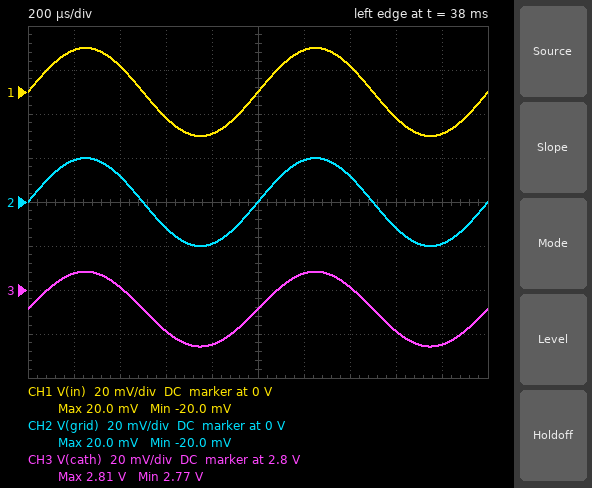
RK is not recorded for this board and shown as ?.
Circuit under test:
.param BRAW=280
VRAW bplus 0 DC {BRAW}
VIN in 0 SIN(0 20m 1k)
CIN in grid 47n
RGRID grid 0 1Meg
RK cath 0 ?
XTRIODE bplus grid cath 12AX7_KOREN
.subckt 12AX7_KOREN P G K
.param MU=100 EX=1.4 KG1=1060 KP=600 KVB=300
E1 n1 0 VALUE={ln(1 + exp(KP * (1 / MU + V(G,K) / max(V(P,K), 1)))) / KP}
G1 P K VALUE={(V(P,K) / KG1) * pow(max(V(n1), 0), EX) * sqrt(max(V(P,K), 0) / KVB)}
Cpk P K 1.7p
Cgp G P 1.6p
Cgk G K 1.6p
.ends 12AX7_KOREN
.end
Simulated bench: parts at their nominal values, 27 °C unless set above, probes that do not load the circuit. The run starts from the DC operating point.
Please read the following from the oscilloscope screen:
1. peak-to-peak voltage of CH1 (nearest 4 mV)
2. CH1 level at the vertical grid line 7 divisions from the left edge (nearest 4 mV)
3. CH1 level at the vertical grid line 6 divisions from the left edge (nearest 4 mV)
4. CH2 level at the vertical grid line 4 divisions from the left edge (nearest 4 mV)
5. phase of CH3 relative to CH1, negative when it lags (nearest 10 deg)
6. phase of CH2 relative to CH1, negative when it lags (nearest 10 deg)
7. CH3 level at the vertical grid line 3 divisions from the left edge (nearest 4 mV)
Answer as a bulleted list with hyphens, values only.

- 40 mV
- 12 mV
- 20 mV
- -20 mV
- 0 deg
- 0 deg
- 2.780 V
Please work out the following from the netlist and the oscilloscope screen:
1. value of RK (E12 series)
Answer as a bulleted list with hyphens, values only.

- 150 kΩ
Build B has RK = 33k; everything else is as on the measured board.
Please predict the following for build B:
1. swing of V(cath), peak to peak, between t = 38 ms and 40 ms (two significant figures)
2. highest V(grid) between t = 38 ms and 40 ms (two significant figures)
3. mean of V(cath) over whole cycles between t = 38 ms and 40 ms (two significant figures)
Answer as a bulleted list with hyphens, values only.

- 30 mV
- 20 mV
- 2.1 V
